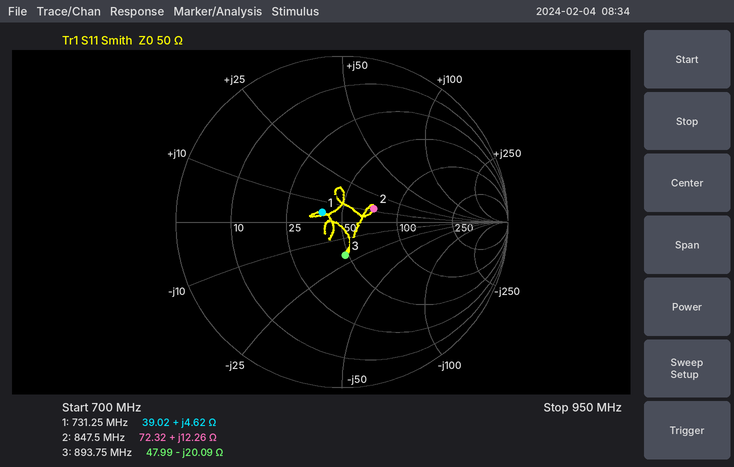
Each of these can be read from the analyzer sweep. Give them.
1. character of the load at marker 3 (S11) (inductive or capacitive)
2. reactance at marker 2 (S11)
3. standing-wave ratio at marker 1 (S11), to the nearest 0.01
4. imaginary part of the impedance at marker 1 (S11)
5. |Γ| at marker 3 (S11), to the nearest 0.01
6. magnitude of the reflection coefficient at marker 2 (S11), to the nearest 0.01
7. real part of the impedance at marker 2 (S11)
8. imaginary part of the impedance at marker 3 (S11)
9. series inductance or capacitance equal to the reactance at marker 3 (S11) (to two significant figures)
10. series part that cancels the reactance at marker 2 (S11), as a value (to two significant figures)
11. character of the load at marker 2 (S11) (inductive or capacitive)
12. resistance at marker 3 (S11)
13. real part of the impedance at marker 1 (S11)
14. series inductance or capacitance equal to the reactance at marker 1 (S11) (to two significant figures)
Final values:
capacitive
+12.26 Ω
1.31
+4.62 Ω
0.20
0.21
72.32 Ω
-20.09 Ω
8.9 pF
15 pF
inductive
47.99 Ω
39.02 Ω
1.0 nH
